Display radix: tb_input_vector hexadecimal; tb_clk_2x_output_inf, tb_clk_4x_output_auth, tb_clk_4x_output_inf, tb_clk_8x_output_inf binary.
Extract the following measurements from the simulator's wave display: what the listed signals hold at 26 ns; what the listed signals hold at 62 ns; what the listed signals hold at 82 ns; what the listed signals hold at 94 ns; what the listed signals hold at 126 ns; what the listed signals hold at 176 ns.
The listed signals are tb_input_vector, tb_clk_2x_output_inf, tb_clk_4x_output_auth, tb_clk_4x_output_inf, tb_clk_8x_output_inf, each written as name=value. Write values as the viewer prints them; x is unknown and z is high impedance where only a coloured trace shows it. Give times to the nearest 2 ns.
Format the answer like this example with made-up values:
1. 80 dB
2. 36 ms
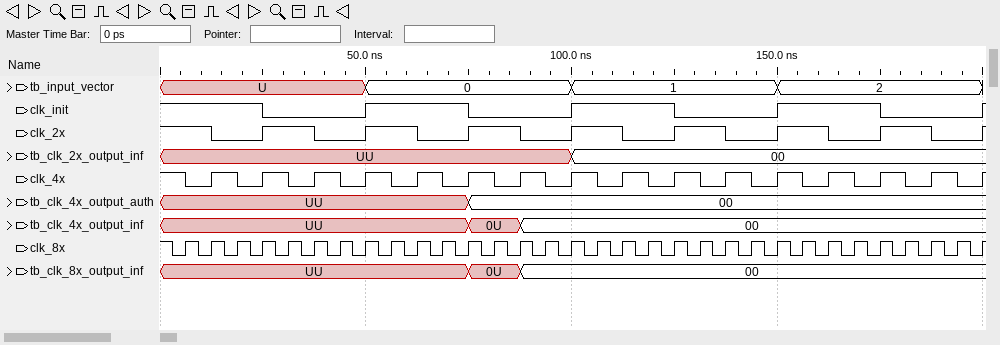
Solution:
1. tb_input_vector=U, tb_clk_2x_output_inf=UU, tb_clk_4x_output_auth=UU, tb_clk_4x_output_inf=UU, tb_clk_8x_output_inf=UU
2. tb_input_vector=0, tb_clk_2x_output_inf=UU, tb_clk_4x_output_auth=UU, tb_clk_4x_output_inf=UU, tb_clk_8x_output_inf=UU
3. tb_input_vector=0, tb_clk_2x_output_inf=UU, tb_clk_4x_output_auth=00, tb_clk_4x_output_inf=0U, tb_clk_8x_output_inf=0U
4. tb_input_vector=0, tb_clk_2x_output_inf=UU, tb_clk_4x_output_auth=00, tb_clk_4x_output_inf=00, tb_clk_8x_output_inf=00
5. tb_input_vector=1, tb_clk_2x_output_inf=00, tb_clk_4x_output_auth=00, tb_clk_4x_output_inf=00, tb_clk_8x_output_inf=00
6. tb_input_vector=2, tb_clk_2x_output_inf=00, tb_clk_4x_output_auth=00, tb_clk_4x_output_inf=00, tb_clk_8x_output_inf=00
